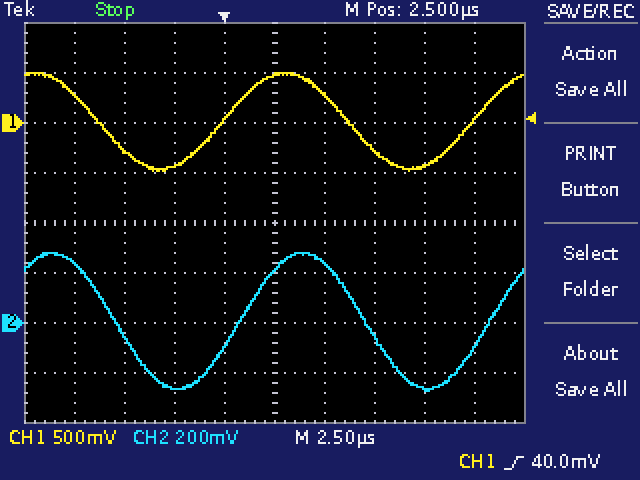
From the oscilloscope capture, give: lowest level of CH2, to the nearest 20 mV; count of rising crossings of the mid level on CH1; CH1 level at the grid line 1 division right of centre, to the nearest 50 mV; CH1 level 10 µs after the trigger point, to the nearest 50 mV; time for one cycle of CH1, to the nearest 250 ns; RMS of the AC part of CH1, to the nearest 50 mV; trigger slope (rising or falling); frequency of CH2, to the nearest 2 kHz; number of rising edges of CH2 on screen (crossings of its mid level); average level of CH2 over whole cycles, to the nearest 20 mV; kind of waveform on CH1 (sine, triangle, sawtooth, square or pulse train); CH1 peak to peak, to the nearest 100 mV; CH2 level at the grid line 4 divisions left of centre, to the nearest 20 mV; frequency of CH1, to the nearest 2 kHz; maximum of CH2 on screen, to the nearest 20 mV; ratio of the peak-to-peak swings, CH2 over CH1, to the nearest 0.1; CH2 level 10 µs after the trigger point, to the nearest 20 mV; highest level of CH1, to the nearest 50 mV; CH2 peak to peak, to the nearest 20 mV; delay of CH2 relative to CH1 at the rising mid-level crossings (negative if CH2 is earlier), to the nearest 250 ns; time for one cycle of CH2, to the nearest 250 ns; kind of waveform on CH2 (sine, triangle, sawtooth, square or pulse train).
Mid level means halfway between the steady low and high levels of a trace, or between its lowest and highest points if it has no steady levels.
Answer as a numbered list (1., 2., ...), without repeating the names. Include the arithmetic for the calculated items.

1. -280 mV
2. 2
3. 300 mV
4. -450 mV
5. 12.50 µs
6. 1.00 V / (2√2) ≈ 354 mV, so 350 mV to the nearest 50 mV
7. rising
8. 1 / 12.50 µs ≈ 80 kHz
9. 2
10. (280 mV + (-280 mV)) / 2 ≈ 0 mV
11. sine
12. 1.00 V
13. 240 mV
14. 1 / 12.50 µs ≈ 80 kHz
15. 280 mV
16. 560 mV / 1.00 V ≈ 0.6
17. -260 mV
18. 500 mV
19. 280 mV − (-280 mV) = 560 mV
20. +750 ns
21. 12.50 µs
22. sine
